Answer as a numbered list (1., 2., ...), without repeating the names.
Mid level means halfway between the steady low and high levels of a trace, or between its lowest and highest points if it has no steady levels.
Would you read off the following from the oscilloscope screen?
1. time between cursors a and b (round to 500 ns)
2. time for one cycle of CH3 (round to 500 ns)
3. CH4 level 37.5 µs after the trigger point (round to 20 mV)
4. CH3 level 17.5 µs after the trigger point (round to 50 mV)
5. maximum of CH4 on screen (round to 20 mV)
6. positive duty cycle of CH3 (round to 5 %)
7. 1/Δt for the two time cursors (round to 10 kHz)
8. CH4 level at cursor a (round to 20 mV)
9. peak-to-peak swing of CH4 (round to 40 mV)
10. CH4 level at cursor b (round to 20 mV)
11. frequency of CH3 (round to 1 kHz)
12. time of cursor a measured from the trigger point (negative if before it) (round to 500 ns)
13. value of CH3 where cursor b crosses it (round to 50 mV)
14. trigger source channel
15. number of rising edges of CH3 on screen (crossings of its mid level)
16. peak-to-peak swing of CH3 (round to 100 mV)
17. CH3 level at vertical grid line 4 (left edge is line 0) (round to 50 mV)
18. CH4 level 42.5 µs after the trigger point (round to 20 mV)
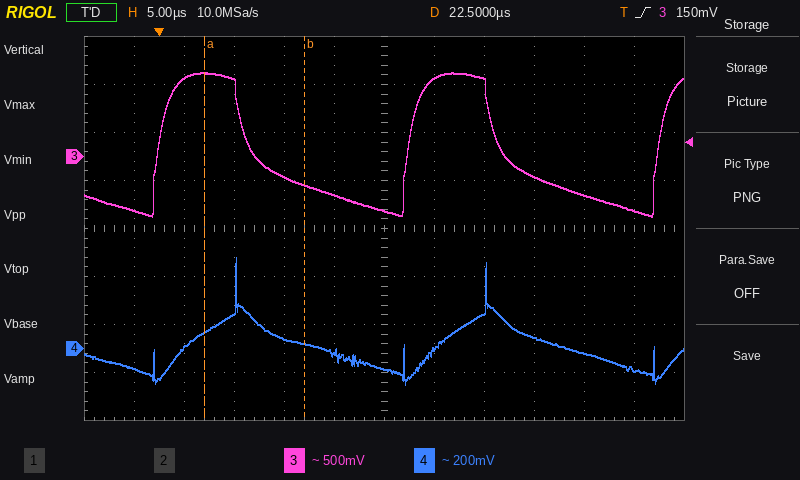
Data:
1. 10.0 µs
2. 25.0 µs
3. 40 mV
4. -400 mV
5. 380 mV
6. 35 %
7. 100 kHz
8. 60 mV
9. 520 mV
10. 20 mV
11. 40 kHz
12. +4.5 µs
13. -300 mV
14. CH3
15. 3
16. 1.50 V
17. -200 mV
18. -20 mV
